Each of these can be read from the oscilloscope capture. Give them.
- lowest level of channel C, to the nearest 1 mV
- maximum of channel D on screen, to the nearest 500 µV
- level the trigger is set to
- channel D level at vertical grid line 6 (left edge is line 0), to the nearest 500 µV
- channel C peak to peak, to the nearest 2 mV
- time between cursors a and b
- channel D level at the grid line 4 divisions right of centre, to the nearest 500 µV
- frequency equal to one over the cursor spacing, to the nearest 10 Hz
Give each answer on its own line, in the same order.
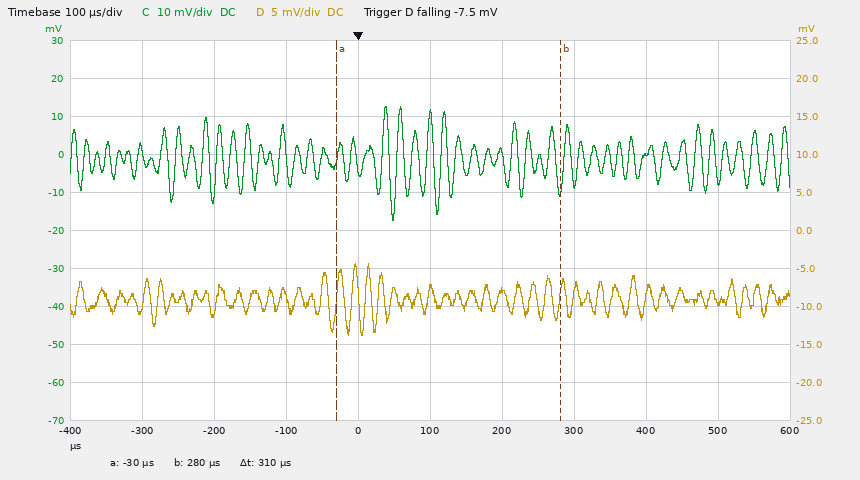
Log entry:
-17 mV
-4.5 mV
-7.5 mV
-8.0 mV
30 mV
310 µs
-9.5 mV
3.23 kHz
